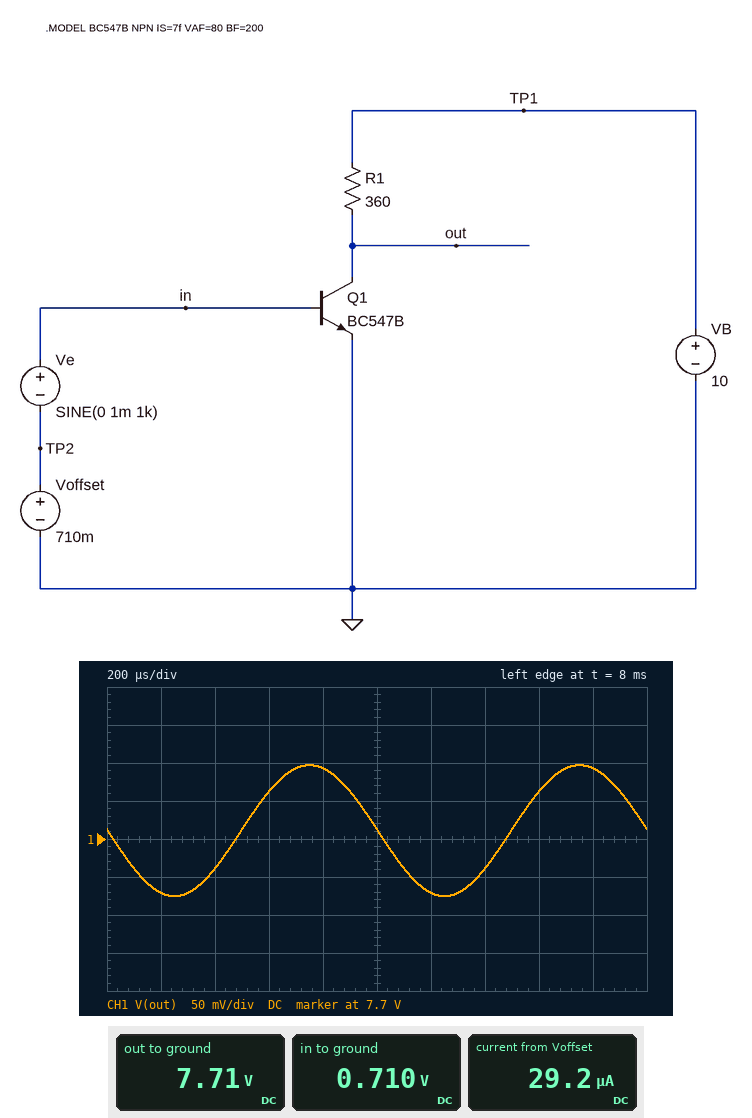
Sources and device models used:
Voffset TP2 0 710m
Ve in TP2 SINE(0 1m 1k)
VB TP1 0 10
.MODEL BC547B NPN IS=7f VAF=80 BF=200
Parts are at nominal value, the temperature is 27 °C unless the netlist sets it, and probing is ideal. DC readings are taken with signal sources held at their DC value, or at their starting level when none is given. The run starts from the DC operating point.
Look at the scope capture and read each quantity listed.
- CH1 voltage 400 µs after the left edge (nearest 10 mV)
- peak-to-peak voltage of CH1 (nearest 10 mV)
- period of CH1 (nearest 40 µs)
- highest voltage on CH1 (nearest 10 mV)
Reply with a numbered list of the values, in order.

1. 7.66 V
2. 170 mV
3. 1.00 ms
4. 7.80 V
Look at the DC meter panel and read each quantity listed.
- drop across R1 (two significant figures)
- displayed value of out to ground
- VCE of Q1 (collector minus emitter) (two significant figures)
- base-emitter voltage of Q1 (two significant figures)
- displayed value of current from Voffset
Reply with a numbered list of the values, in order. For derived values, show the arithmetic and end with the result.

1. 10 V - 7.71 V = 2.3 V
2. 7.71 V
3. 7.71 V = 7.7 V
4. 710 mV = 710 mV
5. 29.2 µA
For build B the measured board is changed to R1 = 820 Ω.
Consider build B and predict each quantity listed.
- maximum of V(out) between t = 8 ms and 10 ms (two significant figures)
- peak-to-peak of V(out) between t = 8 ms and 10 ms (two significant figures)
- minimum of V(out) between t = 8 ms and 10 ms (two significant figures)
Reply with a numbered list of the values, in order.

1. 5.1 V
2. 370 mV
3. 4.8 V
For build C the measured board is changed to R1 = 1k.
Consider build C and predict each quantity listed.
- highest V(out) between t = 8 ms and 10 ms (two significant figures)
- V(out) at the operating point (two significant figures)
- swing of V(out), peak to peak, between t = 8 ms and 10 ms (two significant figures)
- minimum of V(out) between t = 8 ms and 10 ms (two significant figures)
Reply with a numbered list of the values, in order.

1. 4.1 V
2. 3.9 V
3. 440 mV
4. 3.7 V
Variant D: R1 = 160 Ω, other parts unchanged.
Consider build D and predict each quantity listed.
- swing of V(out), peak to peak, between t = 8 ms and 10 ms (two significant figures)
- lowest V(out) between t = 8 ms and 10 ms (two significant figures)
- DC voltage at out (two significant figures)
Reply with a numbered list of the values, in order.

1. 79 mV
2. 8.9 V
3. 9.0 V
